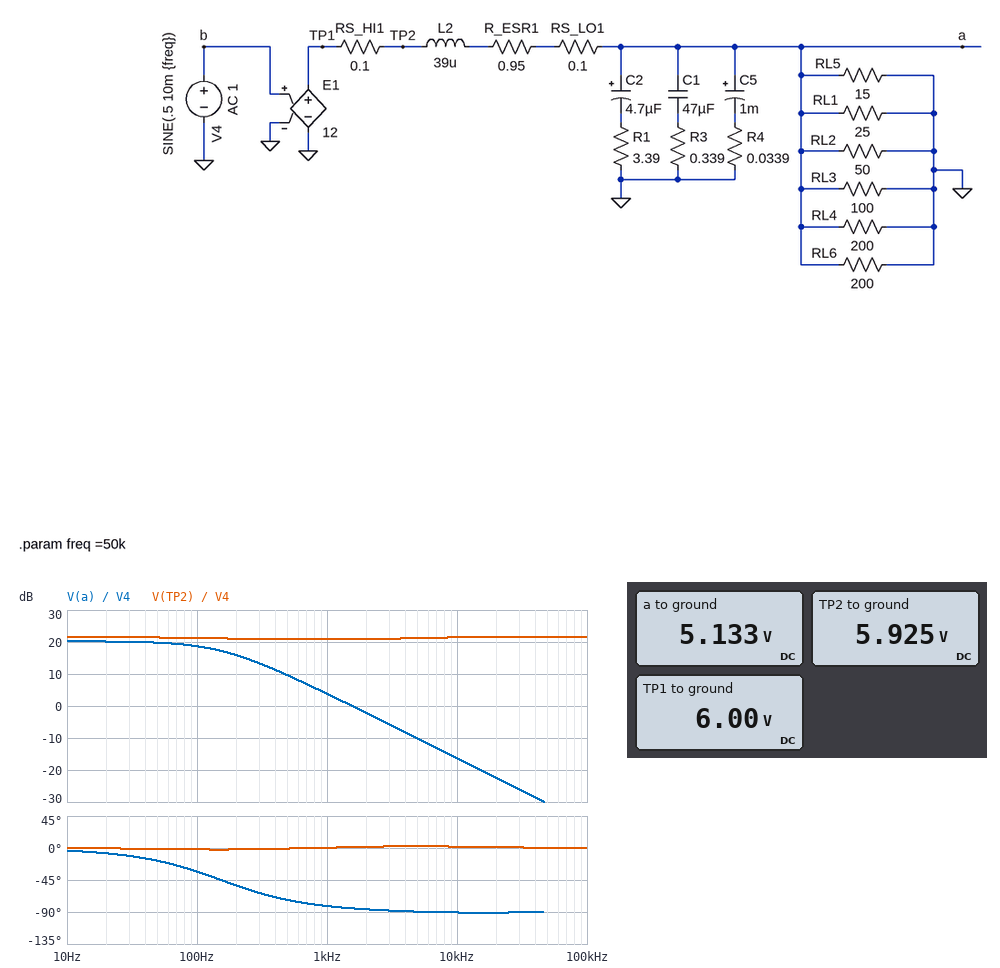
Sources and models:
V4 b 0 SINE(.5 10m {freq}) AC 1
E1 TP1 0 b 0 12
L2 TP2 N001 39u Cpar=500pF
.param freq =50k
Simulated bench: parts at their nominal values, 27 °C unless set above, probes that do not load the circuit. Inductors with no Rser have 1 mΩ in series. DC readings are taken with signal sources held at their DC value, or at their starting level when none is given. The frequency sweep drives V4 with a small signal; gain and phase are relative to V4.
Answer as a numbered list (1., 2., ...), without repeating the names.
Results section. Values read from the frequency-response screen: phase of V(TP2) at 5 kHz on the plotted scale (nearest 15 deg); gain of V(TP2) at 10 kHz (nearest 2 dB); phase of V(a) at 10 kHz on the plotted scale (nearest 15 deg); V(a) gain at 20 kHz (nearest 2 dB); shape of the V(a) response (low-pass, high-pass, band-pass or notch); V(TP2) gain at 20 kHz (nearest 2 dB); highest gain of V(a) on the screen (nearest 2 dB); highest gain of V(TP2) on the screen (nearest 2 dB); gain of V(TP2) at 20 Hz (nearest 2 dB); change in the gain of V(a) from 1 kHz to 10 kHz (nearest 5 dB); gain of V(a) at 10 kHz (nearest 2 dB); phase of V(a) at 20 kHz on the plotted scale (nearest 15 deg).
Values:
1. 0 deg
2. 22 dB
3. -90 deg
4. -22 dB
5. low-pass
6. 22 dB
7. 20 dB
8. 22 dB
9. 22 dB
10. -20 dB
11. -16 dB
12. -90 deg
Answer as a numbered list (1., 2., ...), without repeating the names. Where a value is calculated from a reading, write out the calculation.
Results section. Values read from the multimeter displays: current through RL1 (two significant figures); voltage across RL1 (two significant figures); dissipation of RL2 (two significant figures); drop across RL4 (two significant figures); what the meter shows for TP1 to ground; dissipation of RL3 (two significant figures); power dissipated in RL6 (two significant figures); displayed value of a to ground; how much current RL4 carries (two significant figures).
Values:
1. (5.133 V) / 25 Ω = 210 mA
2. 5.133 V = 5.1 V
3. (5.133 V)^2 / 50 Ω = 530 mW
4. 5.133 V = 5.1 V
5. 6.00 V
6. (5.133 V)^2 / 100 Ω = 260 mW
7. (5.133 V)^2 / 200 Ω = 130 mW
8. 5.133 V
9. (5.133 V) / 200 Ω = 26 mA
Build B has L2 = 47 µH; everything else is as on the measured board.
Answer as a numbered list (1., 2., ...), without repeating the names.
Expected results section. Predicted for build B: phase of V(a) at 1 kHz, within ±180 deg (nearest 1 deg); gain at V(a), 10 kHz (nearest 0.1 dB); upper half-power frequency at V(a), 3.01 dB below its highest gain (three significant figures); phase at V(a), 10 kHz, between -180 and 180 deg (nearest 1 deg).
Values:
1. -84 deg
2. -17.7 dB
3. 154 Hz
4. -95 deg
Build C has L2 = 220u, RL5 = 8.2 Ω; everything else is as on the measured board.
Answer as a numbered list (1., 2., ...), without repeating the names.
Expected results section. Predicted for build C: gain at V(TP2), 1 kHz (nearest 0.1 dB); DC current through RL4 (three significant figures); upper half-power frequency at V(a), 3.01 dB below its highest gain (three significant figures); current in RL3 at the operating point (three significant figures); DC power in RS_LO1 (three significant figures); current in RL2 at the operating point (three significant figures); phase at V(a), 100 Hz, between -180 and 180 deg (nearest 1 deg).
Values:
1. 21.2 dB
2. 24.3 mA
3. 181 Hz
4. 48.7 mA
5. 96.7 mW
6. 97.4 mA
7. -34 deg
